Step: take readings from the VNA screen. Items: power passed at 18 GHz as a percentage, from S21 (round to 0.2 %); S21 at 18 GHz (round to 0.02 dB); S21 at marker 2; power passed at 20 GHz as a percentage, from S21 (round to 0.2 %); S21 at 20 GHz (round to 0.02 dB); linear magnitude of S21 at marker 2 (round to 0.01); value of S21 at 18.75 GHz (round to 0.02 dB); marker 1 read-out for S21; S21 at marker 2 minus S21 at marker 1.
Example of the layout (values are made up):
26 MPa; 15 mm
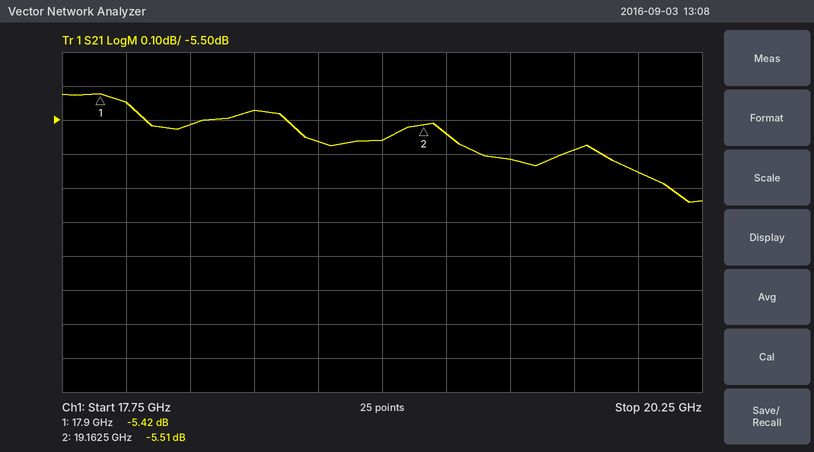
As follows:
28.6 %; -5.44 dB; -5.51 dB; 27.2 %; -5.66 dB; 0.53; -5.56 dB; -5.42 dB; -0.09 dB
